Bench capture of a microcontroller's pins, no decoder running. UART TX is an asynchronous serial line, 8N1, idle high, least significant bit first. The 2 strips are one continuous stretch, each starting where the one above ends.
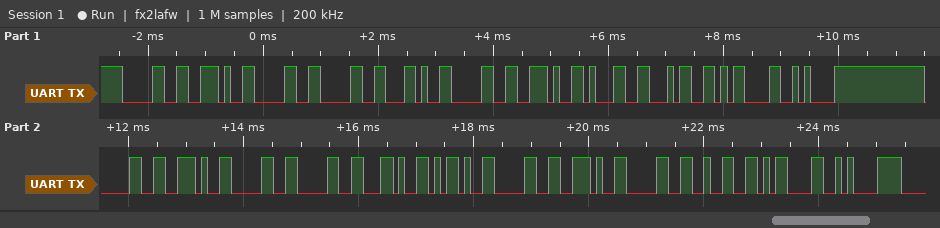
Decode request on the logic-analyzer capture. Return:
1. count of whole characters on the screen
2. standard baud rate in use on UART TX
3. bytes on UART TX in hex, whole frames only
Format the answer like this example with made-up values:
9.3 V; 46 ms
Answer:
23; 9600 baud; 30 2E 30 30 2C 30 2E 31 34 0D 0A 30 2E 30 30 2C 2D 30 2E 30 32 0D 0A
